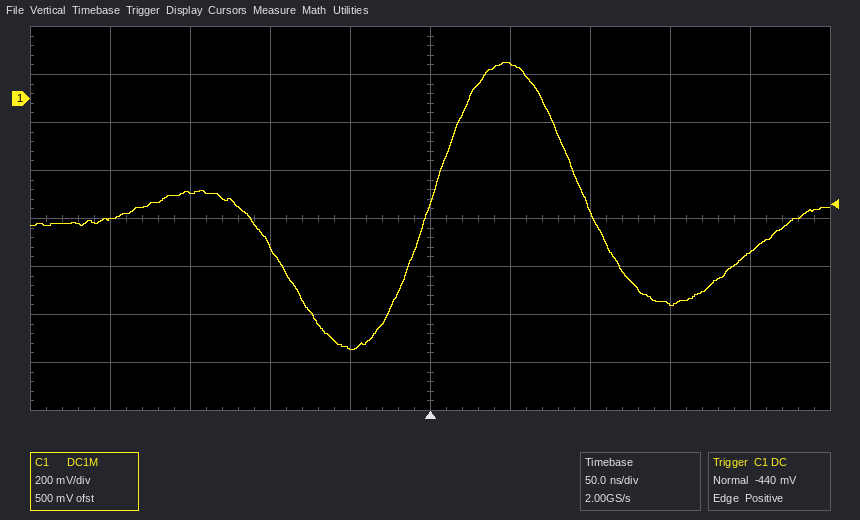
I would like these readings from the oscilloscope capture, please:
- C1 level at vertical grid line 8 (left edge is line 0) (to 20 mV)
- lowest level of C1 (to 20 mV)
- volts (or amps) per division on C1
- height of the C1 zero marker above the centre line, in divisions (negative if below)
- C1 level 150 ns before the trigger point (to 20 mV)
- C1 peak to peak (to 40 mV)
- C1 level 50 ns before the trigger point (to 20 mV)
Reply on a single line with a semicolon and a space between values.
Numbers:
-860 mV; -1.04 V; 200 mV; +2.5 div; -400 mV; 1.20 V; -1.04 V
